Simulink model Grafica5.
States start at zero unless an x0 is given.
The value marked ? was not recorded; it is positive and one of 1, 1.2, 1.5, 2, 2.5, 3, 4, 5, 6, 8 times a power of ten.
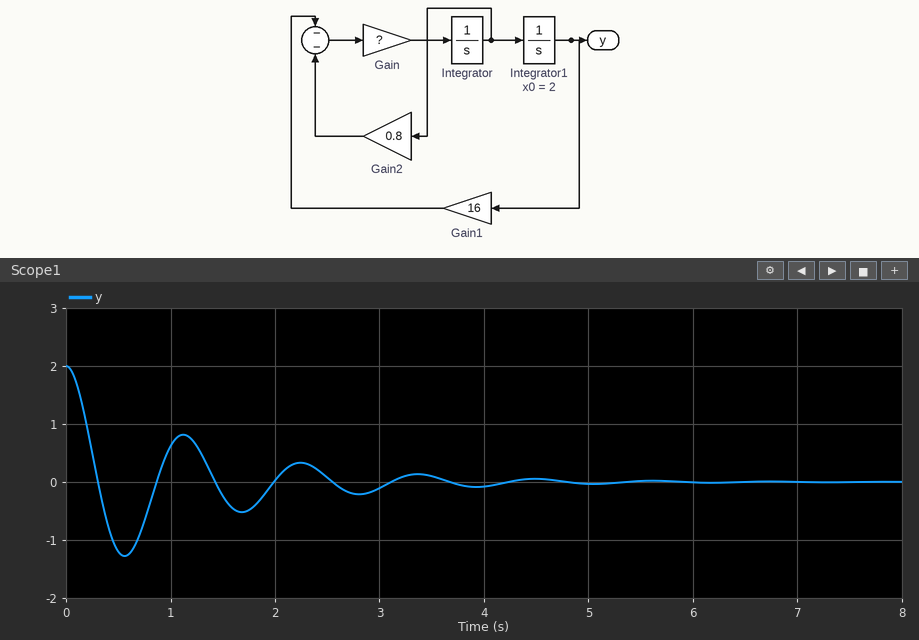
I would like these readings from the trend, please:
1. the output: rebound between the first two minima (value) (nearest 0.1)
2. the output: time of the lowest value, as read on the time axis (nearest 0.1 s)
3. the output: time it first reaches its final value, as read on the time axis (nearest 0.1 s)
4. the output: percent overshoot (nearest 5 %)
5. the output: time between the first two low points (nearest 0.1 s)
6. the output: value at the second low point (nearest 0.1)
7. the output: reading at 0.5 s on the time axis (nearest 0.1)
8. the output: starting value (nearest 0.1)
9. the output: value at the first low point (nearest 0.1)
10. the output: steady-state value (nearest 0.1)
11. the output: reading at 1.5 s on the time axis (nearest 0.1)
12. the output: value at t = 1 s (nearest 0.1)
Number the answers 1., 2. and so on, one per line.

1. 0.8
2. 0.6 s
3. 0.3 s
4. 65 %
5. 1.1 s
6. -0.5
7. -1.2
8. 2.0
9. -1.3
10. 0.0
11. -0.2
12. 0.6
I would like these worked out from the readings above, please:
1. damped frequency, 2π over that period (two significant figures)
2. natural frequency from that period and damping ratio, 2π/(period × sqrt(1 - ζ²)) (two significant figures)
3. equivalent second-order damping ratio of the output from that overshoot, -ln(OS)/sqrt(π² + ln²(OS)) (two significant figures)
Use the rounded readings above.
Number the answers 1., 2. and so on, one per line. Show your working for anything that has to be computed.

1. 2π / 1.1 = 5.7 rad/s
2. 2π / (1.1 × sqrt(1 - 0.14²)) = 5.8 rad/s
3. ln(0.65) = -0.431; 0.431 / sqrt(9.870 + 0.186) = 0.14
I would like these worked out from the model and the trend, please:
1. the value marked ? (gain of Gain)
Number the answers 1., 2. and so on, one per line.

1. 2
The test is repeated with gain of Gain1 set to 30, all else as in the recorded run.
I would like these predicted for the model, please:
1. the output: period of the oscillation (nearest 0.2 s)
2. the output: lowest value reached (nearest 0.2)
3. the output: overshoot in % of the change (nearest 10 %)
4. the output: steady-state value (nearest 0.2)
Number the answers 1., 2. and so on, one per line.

1. 0.8 s
2. -1.4
3. 70 %
4. 0.0
